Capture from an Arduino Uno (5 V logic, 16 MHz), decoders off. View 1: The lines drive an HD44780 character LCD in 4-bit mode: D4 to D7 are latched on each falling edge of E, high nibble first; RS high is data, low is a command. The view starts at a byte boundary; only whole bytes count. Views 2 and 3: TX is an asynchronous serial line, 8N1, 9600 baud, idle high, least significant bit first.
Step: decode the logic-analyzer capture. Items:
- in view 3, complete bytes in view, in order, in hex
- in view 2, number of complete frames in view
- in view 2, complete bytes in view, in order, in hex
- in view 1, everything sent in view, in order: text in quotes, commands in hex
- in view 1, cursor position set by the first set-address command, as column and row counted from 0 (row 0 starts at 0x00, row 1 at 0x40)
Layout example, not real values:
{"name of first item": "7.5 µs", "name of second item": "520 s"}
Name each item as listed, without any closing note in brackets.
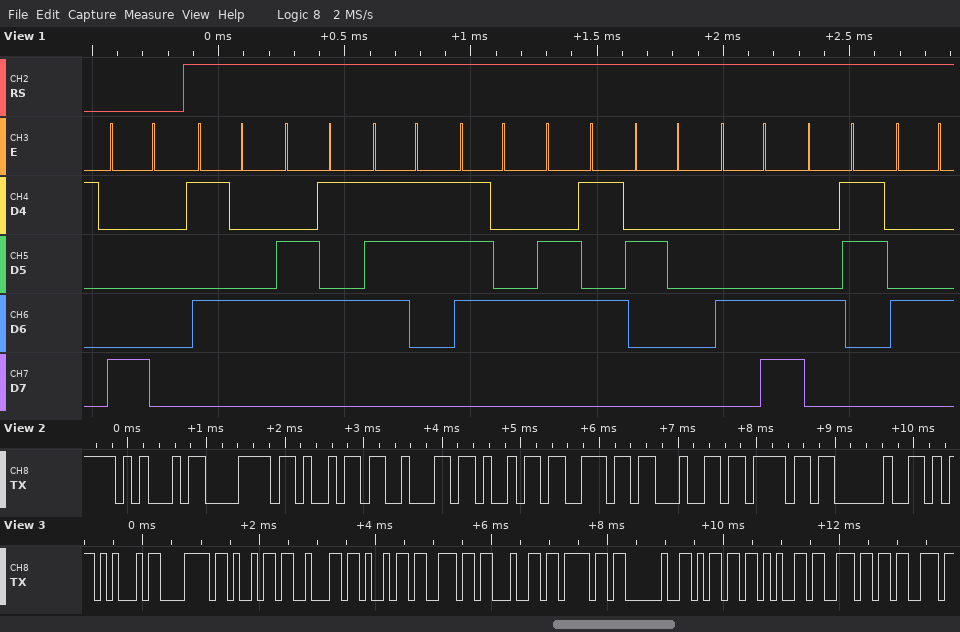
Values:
{"in view 3, complete bytes in view, in order, in hex": "45 78 69 62 69 6E 64 6F 20 6D 65 6E 73", "in view 2, number of complete frames in view": "9", "in view 2, complete bytes in view, in order, in hex": "45 78 69 62 69 6E 64 6F 20", "in view 1, everything sent in view, in order: text in quotes, commands in hex": "0x80 \"Teste LCD\"", "in view 1, cursor position set by the first set-address command, as column and row counted from 0": "column 0, row 0"}
